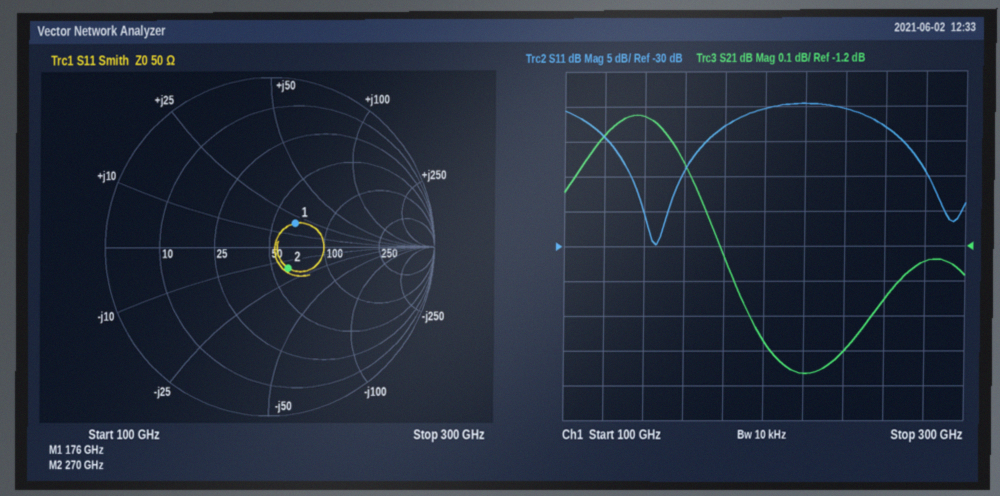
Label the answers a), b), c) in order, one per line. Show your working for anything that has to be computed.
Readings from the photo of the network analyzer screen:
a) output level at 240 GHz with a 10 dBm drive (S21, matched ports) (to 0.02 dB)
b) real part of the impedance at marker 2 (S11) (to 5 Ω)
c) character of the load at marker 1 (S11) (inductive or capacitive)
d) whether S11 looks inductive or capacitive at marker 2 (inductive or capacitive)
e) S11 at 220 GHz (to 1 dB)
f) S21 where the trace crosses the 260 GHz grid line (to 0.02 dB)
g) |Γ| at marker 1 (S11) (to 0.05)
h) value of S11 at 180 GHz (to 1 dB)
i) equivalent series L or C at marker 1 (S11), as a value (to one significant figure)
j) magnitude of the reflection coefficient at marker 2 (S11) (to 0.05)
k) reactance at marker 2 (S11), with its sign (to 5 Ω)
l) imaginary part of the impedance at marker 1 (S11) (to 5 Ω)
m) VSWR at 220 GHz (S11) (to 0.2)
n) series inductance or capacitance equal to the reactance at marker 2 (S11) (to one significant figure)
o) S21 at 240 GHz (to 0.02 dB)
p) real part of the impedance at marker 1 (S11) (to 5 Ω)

a) 10 dBm + (-1.50 dB) = 8.50 dBm
b) 60 Ω
c) inductive
d) capacitive
e) -10 dB
f) -1.36 dB
g) 0.20
h) -13 dB
i) L = 20 Ω/(2π × 176 GHz) ≈ 18.1 pH, so 20 pH to one significant figure
j) 0.15
k) -15 Ω
l) +20 Ω
m) |Γ| = 10^(-10/20) = 0.3162; VSWR = (1 + 0.3162)/(1 − 0.3162) ≈ 1.92, so 2.0 to the nearest 0.2
n) C = 1/(2π × 270 GHz × 15 Ω) ≈ 39.3 fF, so 40 fF to one significant figure
o) -1.50 dB
p) 65 Ω
